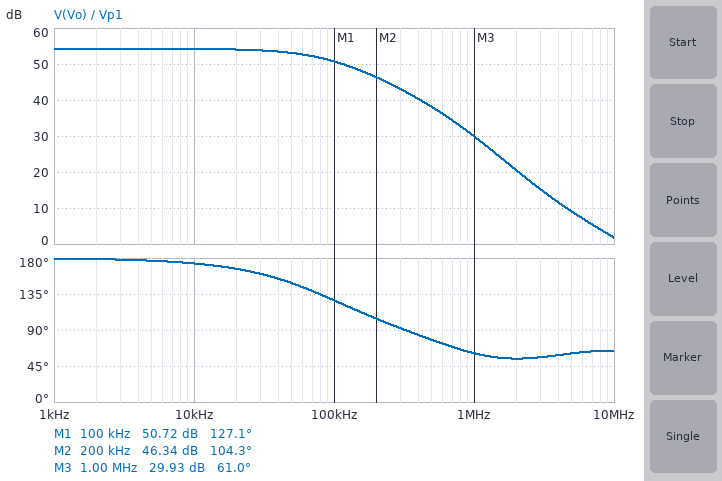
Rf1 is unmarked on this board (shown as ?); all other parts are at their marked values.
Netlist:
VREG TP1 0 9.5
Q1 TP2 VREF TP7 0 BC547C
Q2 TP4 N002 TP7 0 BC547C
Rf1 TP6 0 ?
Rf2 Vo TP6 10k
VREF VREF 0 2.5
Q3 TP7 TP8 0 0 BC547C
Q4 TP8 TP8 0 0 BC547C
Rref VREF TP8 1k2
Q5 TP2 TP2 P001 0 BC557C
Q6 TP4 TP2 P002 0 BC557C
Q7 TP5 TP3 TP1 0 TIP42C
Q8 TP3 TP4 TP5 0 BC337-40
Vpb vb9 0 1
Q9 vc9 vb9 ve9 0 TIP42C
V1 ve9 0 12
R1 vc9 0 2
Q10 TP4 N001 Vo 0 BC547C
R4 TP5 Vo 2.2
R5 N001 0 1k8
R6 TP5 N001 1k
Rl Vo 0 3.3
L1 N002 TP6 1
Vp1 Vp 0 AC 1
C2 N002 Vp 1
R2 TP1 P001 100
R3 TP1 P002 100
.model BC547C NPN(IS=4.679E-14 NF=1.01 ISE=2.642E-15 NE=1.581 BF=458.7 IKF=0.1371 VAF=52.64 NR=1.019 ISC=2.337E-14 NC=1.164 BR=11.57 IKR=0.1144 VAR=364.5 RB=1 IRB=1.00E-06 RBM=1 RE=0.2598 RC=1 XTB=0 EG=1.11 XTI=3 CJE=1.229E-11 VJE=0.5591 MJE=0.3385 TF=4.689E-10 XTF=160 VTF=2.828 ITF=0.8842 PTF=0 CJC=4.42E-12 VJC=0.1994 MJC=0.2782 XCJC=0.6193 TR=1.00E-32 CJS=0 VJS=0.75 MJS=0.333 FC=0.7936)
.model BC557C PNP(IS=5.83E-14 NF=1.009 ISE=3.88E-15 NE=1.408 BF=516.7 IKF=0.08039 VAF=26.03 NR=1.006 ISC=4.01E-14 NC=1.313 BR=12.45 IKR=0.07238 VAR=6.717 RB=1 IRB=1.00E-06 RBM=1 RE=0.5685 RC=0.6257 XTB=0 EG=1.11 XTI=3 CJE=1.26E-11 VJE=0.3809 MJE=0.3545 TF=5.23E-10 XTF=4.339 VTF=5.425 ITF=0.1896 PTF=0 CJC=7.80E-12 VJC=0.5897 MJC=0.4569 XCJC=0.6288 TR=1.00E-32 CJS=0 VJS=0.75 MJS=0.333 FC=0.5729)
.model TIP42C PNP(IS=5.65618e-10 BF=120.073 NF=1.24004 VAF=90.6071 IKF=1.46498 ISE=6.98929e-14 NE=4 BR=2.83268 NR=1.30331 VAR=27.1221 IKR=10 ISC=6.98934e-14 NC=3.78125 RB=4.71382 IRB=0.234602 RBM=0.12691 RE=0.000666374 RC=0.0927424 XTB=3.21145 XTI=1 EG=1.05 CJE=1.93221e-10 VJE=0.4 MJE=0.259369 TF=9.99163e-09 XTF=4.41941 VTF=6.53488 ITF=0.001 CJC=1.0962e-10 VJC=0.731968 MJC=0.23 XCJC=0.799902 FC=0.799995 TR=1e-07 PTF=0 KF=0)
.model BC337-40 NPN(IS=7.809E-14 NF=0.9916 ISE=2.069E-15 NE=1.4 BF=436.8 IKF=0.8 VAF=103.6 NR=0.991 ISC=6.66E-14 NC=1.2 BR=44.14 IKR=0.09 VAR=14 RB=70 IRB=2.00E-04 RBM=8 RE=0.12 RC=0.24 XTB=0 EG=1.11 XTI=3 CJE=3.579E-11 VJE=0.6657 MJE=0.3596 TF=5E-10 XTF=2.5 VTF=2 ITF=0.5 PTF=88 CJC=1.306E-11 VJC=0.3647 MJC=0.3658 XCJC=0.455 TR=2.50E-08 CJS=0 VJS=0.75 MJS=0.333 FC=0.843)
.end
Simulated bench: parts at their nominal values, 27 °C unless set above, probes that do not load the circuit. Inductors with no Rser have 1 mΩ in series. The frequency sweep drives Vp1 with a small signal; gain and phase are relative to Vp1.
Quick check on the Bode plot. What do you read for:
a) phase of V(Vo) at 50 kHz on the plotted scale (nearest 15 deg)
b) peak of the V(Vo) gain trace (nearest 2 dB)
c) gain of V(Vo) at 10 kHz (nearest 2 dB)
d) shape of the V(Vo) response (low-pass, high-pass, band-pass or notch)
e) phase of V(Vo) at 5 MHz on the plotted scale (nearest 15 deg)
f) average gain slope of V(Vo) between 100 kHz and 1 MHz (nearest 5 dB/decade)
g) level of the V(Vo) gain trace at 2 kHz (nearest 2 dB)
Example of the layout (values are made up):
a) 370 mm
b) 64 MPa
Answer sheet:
a) 150 deg
b) 54 dB
c) 54 dB
d) low-pass
e) 60 deg
f) -20 dB/decade
g) 54 dB
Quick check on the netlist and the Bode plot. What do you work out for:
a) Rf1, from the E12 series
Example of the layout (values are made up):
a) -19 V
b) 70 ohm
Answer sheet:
a) 12 kΩ
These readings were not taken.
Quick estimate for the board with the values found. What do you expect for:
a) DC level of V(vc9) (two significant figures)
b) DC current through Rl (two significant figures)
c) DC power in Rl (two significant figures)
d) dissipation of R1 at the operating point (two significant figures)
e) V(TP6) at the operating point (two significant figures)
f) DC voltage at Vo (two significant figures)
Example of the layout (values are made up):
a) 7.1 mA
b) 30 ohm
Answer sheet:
a) 11 V
b) 1.4 A
c) 6.4 W
d) 65 W
e) 2.5 V
f) 4.6 V
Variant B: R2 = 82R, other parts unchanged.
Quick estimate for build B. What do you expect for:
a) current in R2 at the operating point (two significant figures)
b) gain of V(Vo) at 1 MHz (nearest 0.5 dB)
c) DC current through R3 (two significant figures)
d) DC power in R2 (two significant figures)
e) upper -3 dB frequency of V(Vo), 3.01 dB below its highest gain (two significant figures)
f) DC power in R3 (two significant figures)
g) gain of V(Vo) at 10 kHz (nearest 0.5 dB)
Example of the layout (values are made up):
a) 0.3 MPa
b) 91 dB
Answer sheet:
a) 880 µA
b) 29.0 dB
c) 760 µA
d) 63 µW
e) 88 kHz
f) 58 µW
g) 53.5 dB
